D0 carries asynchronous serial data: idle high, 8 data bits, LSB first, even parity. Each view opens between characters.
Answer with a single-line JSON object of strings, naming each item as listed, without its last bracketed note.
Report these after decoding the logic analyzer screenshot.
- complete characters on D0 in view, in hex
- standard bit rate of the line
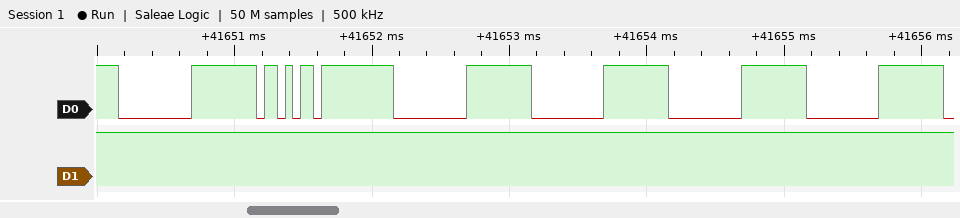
{"complete characters on D0 in view, in hex": "00, 6B, 00, 00, 00, 00", "standard bit rate of the line": "19200 baud"}
